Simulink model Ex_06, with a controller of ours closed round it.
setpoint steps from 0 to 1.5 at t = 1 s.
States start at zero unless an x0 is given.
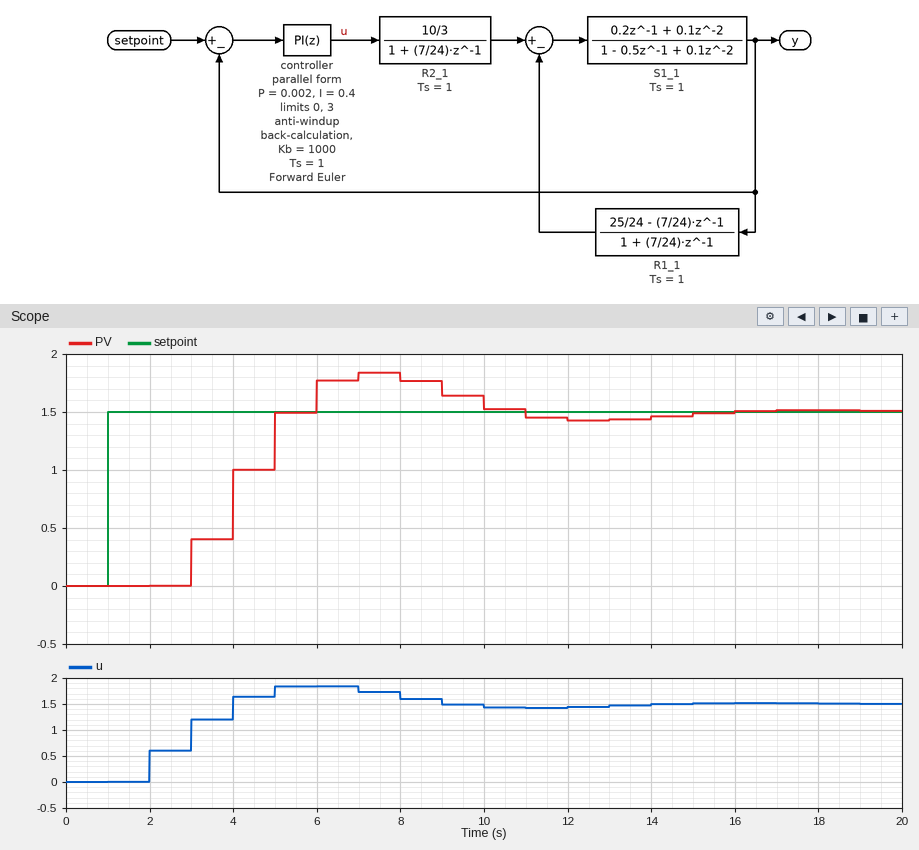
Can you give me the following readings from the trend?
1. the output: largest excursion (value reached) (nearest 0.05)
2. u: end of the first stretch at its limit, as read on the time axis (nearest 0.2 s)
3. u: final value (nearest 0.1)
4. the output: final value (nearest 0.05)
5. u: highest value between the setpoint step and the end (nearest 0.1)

1.85
2.0 s
1.5
1.50
1.8
